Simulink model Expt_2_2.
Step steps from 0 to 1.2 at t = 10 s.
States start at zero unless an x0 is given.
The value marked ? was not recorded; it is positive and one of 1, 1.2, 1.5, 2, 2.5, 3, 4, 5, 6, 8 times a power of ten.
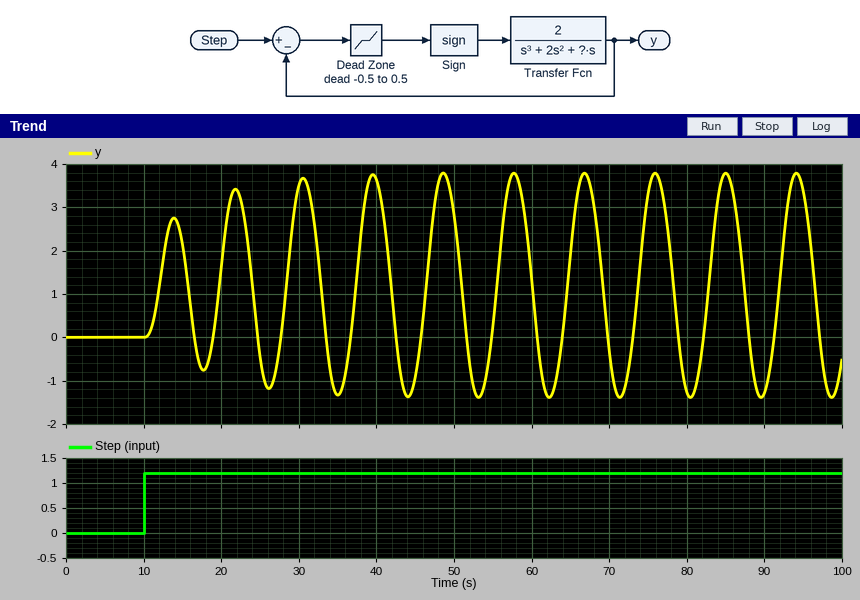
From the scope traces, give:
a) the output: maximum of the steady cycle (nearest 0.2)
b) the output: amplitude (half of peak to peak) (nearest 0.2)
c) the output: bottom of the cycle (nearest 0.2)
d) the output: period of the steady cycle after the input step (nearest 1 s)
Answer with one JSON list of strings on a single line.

["3.8", "2.6", "-1.4", "9 s"]
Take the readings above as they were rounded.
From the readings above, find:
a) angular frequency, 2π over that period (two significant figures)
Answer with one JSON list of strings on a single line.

["0.70 rad/s"]
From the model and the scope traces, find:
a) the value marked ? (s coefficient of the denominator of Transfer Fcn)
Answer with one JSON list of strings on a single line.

["0.5"]
